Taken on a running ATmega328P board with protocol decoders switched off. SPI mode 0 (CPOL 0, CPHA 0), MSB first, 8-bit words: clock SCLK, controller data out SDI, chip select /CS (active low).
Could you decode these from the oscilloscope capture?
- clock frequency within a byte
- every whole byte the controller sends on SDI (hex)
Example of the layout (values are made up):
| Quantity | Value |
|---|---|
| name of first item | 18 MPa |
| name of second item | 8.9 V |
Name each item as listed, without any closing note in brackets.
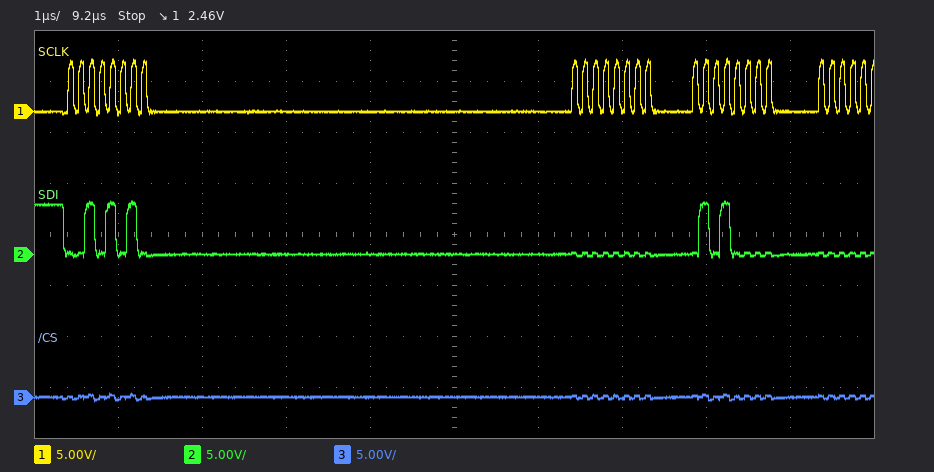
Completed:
| Quantity | Value |
|---|---|
| clock frequency within a byte | 8 MHz |
| every whole byte the controller sends on SDI | 2A 00 50 |
